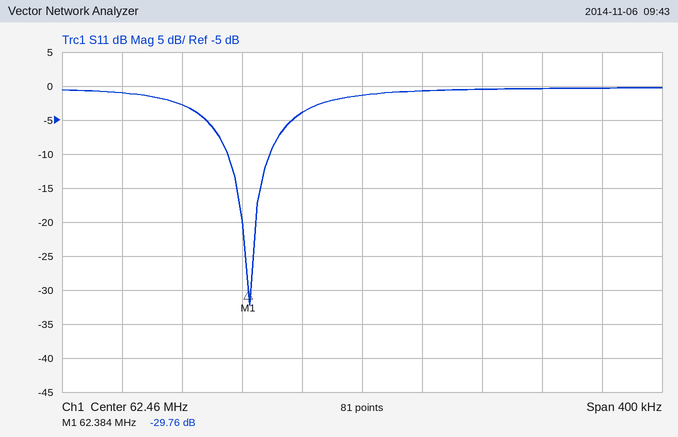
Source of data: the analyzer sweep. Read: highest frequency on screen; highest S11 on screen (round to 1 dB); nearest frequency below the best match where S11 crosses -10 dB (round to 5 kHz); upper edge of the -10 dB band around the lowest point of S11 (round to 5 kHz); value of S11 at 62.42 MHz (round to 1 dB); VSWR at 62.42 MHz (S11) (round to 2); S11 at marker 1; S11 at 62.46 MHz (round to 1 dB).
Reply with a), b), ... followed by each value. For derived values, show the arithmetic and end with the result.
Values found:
a) 62.66 MHz
b) 0 dB
c) 62.370 MHz
d) 62.400 MHz
e) -4 dB
f) |Γ| = 10^(-4/20) = 0.6310; VSWR = (1 + 0.6310)/(1 − 0.6310) ≈ 4
g) -29.76 dB
h) -1 dB
